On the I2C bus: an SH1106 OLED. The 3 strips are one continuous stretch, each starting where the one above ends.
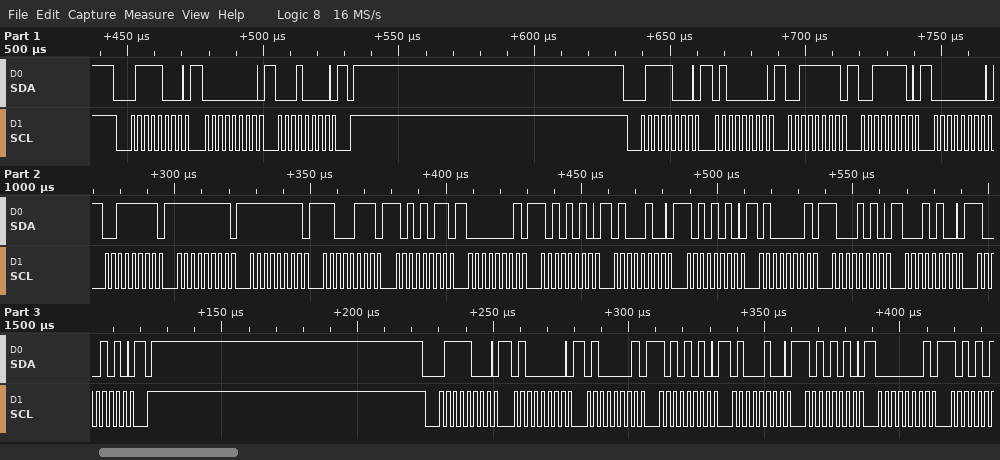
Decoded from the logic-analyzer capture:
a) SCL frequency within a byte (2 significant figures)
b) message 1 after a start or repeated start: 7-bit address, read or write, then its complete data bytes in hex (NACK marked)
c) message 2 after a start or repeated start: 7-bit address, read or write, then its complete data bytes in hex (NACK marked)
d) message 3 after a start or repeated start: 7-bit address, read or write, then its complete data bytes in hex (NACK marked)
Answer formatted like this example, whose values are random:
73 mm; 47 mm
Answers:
400 kHz; 0x3C write: 00 10; 0x3C write: 40 3F 3E 00 3F FF FF C7 AB 01 AA 44 AA 41 8A 14 8A; 0x3C write: 40 41 AA 44 AA 01
